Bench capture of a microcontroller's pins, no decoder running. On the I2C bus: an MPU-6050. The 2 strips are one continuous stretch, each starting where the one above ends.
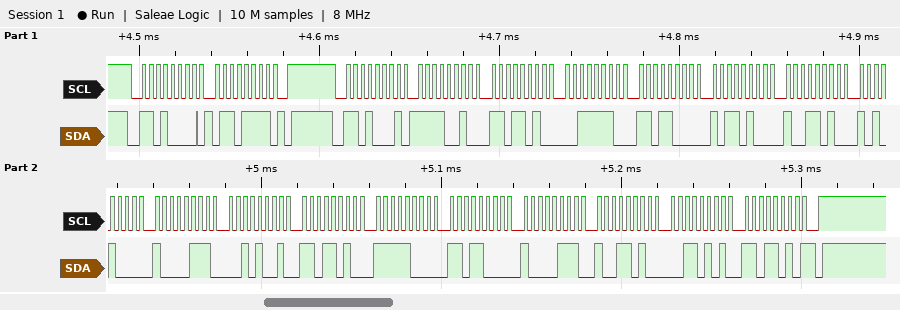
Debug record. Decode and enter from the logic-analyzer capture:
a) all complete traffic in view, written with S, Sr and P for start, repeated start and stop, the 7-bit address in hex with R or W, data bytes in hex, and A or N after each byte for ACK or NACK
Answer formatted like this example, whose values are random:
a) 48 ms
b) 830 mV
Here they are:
a) S 68W A 6F A P S 68R A F2 A DA A 3E A D8 A B4 A 9A A A8 A 87 A 29 A DA A F8 A D8 A 87 A 9A A 35 A DA N P
